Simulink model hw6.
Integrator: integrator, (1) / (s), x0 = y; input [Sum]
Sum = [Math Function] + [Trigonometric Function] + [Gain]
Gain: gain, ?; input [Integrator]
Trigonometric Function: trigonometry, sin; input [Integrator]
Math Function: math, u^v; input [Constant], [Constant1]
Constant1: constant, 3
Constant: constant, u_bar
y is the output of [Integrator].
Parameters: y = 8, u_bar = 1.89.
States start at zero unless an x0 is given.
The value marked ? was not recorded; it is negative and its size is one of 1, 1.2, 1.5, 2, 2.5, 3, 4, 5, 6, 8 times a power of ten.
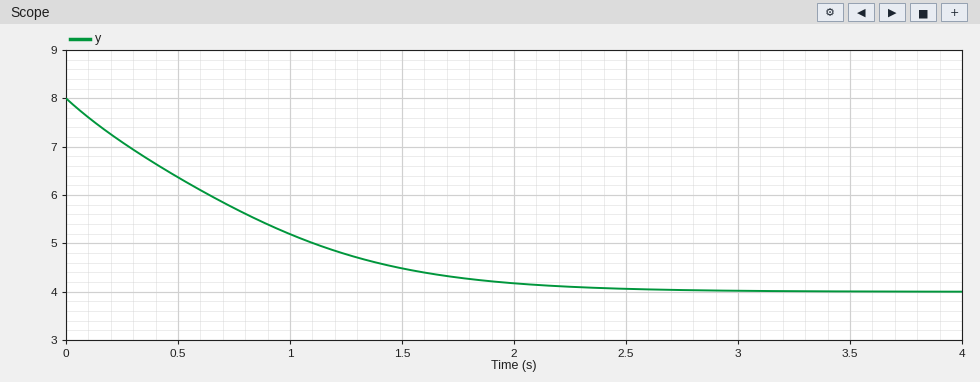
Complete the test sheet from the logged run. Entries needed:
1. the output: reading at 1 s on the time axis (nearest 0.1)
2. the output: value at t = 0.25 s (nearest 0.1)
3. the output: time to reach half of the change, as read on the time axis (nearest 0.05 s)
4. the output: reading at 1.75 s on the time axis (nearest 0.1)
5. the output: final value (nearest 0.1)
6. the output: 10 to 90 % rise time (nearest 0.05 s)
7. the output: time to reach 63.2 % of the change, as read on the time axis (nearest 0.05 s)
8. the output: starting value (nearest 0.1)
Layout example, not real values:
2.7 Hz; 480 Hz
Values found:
5.2; 7.1; 0.65 s; 4.3; 4.0; 1.50 s; 0.85 s; 8.0
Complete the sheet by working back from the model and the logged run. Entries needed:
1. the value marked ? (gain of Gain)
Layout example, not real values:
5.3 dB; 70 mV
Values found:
-1.5
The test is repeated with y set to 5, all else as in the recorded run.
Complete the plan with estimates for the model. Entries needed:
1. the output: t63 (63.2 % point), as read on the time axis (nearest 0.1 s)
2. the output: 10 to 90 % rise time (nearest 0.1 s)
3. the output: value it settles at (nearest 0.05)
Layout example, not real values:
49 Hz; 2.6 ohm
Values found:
0.5 s; 1.1 s; 4.00
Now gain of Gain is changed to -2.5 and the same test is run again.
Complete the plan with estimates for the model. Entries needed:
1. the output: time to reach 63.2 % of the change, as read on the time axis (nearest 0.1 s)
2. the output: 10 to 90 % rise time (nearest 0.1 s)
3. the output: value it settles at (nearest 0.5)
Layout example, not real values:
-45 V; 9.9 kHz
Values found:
0.4 s; 0.7 s; 3.0
